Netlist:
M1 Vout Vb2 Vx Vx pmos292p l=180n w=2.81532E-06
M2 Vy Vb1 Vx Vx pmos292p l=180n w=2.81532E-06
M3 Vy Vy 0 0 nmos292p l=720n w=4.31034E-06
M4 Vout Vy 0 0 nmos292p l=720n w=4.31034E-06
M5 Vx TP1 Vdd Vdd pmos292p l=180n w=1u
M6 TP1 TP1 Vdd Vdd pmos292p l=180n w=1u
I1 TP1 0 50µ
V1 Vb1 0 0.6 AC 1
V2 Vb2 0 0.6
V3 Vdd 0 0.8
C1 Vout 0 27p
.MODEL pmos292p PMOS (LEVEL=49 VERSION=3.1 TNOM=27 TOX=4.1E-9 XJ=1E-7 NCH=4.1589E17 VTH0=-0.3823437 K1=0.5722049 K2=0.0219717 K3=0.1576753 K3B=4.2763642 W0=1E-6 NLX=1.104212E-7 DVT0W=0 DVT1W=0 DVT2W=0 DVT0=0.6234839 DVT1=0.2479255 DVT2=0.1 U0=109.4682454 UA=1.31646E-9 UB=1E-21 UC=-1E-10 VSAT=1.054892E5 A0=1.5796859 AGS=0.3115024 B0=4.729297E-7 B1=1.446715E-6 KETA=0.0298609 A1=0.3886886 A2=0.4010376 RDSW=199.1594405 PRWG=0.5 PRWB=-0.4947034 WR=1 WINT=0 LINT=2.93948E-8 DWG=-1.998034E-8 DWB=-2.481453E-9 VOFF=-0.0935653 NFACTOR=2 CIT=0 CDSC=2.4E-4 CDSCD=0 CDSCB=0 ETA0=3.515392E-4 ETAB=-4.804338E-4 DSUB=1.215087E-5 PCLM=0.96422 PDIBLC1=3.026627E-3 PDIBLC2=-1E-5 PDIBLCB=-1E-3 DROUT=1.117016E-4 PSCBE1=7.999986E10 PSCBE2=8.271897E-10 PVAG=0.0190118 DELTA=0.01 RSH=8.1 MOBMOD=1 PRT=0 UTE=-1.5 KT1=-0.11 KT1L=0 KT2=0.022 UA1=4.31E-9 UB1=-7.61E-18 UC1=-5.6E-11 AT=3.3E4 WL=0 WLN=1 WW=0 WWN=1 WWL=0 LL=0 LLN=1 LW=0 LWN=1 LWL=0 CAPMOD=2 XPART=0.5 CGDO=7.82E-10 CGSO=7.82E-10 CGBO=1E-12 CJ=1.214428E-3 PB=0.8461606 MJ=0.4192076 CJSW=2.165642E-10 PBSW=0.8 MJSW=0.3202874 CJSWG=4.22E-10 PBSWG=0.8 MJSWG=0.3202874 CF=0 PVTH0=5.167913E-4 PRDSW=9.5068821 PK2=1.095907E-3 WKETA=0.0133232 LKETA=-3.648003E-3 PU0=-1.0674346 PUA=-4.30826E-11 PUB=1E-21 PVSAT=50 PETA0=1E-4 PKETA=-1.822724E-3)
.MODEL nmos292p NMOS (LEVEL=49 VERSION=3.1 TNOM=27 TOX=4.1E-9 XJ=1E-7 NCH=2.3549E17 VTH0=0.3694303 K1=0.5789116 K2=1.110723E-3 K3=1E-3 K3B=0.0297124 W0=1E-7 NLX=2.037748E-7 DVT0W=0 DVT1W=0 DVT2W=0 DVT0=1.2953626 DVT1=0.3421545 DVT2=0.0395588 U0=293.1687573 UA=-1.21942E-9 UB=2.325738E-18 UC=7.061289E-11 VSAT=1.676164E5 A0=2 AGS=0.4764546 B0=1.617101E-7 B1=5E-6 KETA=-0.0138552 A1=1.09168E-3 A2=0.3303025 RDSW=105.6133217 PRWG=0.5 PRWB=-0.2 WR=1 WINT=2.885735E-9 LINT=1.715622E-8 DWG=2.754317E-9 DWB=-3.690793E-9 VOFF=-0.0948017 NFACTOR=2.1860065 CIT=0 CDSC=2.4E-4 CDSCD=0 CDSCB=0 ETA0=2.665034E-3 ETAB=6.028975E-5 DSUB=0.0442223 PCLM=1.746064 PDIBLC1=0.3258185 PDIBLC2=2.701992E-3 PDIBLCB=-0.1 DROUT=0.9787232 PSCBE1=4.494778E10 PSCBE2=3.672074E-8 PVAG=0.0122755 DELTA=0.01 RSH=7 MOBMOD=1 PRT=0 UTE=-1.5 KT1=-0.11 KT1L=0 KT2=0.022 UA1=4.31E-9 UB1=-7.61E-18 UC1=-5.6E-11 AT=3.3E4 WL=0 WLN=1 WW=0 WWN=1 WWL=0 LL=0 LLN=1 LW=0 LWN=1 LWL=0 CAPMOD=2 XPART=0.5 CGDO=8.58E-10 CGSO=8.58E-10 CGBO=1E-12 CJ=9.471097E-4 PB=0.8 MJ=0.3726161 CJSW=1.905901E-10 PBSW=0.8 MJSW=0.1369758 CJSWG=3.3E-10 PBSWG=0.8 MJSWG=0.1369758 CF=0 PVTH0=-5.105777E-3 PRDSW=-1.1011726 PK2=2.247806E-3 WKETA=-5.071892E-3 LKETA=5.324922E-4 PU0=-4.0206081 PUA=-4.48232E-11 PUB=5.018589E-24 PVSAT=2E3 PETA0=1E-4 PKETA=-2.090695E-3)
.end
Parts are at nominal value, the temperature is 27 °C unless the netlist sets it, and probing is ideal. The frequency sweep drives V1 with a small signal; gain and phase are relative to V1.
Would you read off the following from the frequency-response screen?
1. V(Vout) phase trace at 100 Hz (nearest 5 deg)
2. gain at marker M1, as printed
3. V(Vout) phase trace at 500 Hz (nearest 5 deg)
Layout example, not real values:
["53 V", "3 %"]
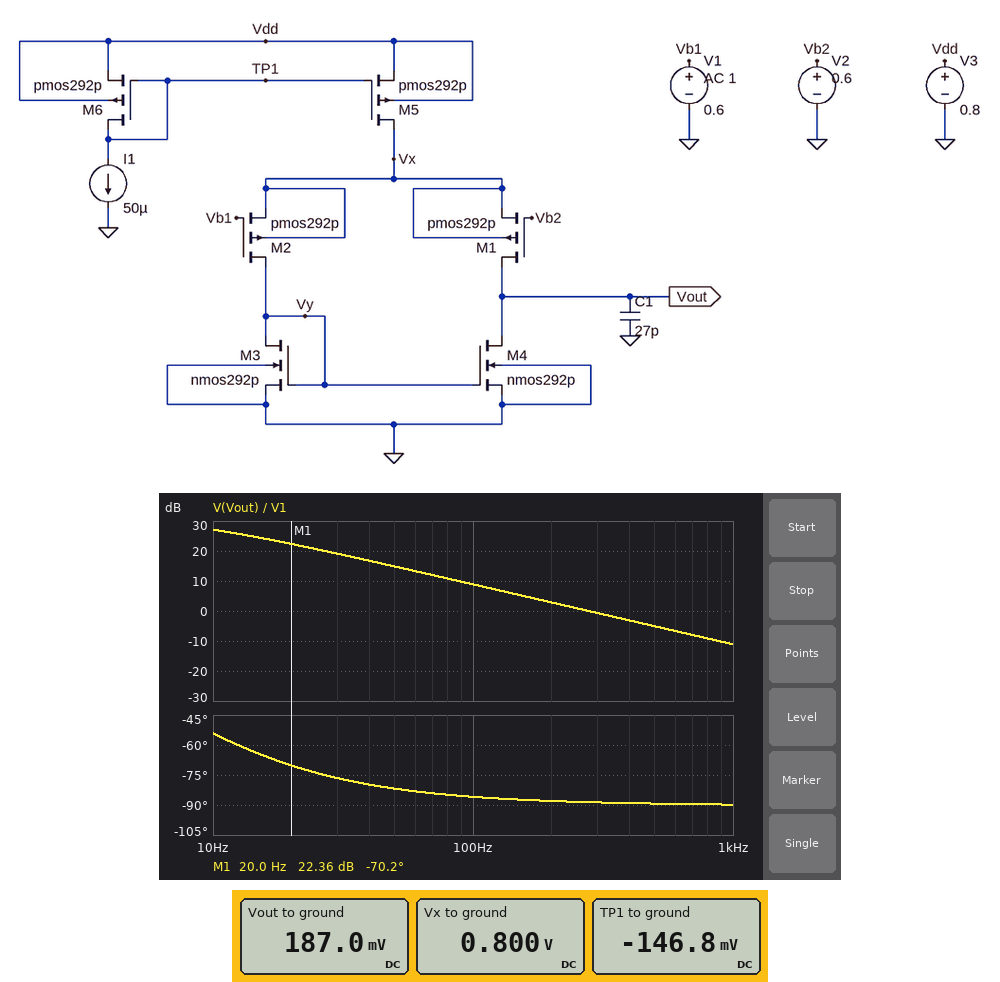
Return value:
["-85 deg", "22.36 dB", "-90 deg"]
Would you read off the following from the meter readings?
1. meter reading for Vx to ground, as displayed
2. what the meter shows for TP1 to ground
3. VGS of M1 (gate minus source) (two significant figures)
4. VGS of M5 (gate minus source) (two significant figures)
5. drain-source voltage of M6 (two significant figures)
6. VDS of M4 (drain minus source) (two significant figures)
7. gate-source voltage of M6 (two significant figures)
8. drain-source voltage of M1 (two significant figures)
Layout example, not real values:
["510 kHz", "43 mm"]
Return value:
["0.800 V", "-146.8 mV", "-200 mV", "-950 mV", "-950 mV", "190 mV", "-950 mV", "-610 mV"]
